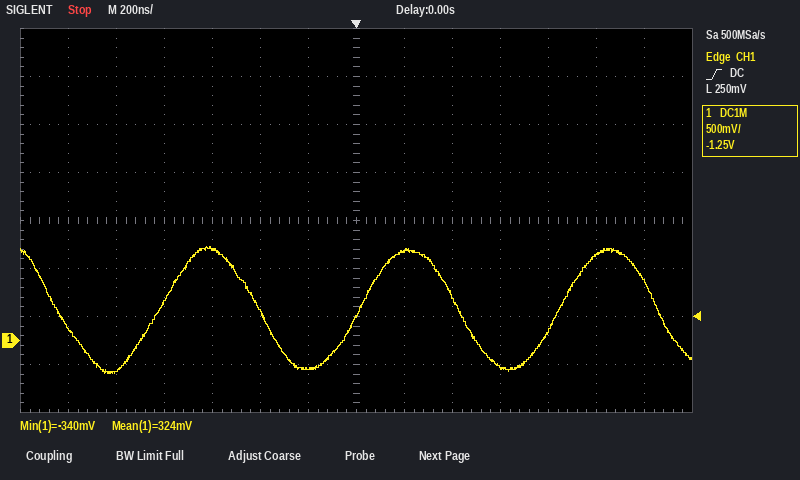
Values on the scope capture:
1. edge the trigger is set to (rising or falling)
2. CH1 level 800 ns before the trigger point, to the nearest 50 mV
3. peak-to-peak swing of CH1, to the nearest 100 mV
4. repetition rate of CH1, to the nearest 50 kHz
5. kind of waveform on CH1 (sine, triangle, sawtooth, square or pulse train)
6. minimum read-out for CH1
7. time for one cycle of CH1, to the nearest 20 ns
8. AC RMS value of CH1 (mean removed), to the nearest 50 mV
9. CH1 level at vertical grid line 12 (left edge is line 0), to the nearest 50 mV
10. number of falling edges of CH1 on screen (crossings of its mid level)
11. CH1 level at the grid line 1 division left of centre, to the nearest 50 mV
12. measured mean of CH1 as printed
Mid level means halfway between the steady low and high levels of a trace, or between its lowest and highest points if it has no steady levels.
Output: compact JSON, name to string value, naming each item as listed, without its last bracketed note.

{"edge the trigger is set to": "rising", "CH1 level 800 ns before the trigger point, to the nearest 50 mV": "400 mV", "peak-to-peak swing of CH1, to the nearest 100 mV": "1.30 V", "repetition rate of CH1, to the nearest 50 kHz": "1.20 MHz", "kind of waveform on CH1": "sine", "minimum read-out for CH1": "-340 mV", "time for one cycle of CH1, to the nearest 20 ns": "840 ns", "AC RMS value of CH1 (mean removed), to the nearest 50 mV": "450 mV", "CH1 level at vertical grid line 12 (left edge is line 0), to the nearest 50 mV": "900 mV", "number of falling edges of CH1 on screen": "4", "CH1 level at the grid line 1 division left of centre, to the nearest 50 mV": "-300 mV", "measured mean of CH1 as printed": "324 mV"}
